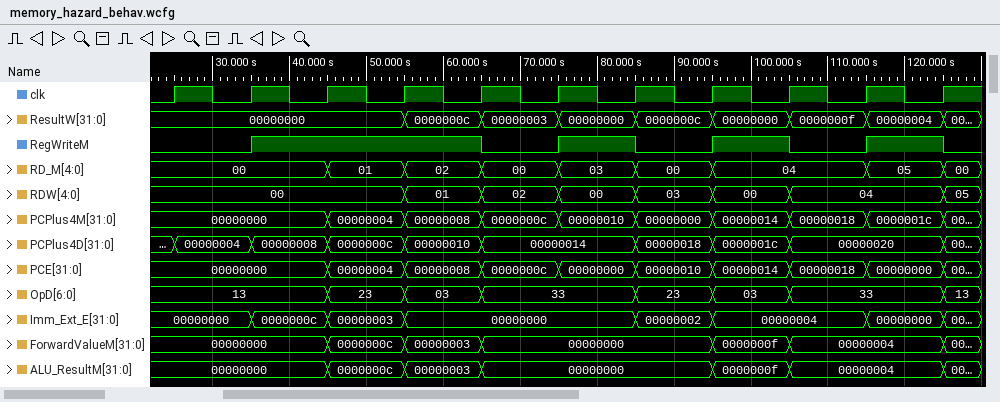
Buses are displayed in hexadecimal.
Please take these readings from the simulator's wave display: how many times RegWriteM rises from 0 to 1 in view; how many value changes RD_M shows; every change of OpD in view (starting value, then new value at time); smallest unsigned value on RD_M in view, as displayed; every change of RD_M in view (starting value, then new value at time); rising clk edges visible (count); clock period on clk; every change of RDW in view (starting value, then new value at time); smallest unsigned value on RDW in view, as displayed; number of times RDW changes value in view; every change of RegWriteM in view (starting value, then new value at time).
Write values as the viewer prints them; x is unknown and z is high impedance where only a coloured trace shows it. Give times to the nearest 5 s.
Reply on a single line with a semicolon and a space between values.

4; 8; 13, 23 at 45 s, 03 at 55 s, 33 at 65 s, 23 at 85 s, 03 at 95 s, 33 at 105 s, 13 at 125 s; 00; 00, 01 at 45 s, 02 at 55 s, 00 at 65 s, 03 at 75 s, 00 at 85 s, 04 at 95 s, 05 at 115 s, 00 at 125 s; 11; 10 s; 00, 01 at 55 s, 02 at 65 s, 00 at 75 s, 03 at 85 s, 00 at 95 s, 04 at 105 s, 05 at 125 s; 00; 7; 0, 1 at 35 s, 0 at 65 s, 1 at 75 s, 0 at 85 s, 1 at 95 s, 0 at 105 s, 1 at 115 s, 0 at 125 s
